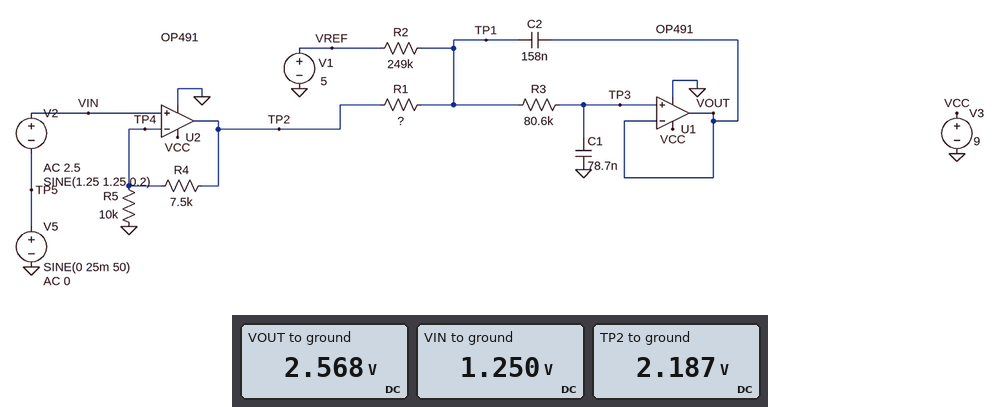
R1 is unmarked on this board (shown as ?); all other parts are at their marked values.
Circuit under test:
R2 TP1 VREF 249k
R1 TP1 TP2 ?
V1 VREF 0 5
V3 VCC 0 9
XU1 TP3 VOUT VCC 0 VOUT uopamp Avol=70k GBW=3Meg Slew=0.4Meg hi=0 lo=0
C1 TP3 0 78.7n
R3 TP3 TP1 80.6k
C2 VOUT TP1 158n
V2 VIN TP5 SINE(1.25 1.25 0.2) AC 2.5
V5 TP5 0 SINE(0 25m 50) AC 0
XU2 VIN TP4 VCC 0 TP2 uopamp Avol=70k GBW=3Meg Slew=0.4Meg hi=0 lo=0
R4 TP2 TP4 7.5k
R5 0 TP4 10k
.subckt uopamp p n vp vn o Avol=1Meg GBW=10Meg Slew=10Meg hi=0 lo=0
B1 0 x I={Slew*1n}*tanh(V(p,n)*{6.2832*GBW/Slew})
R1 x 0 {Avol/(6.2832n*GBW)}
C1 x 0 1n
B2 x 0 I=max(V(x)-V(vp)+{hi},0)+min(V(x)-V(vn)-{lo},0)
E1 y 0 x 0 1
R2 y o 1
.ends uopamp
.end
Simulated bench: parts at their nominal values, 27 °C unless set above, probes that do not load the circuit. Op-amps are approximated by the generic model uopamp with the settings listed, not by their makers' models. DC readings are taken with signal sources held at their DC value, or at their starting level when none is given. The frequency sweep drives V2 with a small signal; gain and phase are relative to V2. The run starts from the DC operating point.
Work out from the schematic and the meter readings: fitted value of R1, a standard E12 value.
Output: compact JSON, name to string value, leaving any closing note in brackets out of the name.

{"fitted value of R1, a standard E12 value": "39 kΩ"}
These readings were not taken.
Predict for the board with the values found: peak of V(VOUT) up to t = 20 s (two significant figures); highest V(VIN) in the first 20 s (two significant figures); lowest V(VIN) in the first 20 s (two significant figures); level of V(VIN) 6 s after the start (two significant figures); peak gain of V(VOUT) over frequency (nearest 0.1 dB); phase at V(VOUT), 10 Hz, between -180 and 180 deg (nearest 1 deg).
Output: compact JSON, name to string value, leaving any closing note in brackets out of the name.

{"peak of V(VOUT) up to t = 20 s": "4.5 V", "highest V(VIN) in the first 20 s": "2.5 V", "lowest V(VIN) in the first 20 s": "-25 mV", "level of V(VIN) 6 s after the start": "2.4 V", "peak gain of V(VOUT) over frequency": "3.6 dB", "phase at V(VOUT), 10 Hz, between -180 and 180 deg": "-33 deg"}
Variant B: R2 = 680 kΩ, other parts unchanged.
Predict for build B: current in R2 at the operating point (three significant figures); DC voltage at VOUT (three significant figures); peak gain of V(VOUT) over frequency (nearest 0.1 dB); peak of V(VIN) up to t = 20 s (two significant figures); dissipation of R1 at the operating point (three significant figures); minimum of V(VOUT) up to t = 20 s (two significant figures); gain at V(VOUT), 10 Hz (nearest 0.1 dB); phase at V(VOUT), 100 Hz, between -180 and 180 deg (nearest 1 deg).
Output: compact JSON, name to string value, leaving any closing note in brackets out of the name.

{"current in R2 at the operating point": "3.91 µA", "DC voltage at VOUT": "2.34 V", "peak gain of V(VOUT) over frequency": "4.4 dB", "peak of V(VIN) up to t = 20 s": "2.5 V", "dissipation of R1 at the operating point": "597 nW", "minimum of V(VOUT) up to t = 20 s": "280 mV", "gain at V(VOUT), 10 Hz": "4.1 dB", "phase at V(VOUT), 100 Hz, between -180 and 180 deg": "-157 deg"}
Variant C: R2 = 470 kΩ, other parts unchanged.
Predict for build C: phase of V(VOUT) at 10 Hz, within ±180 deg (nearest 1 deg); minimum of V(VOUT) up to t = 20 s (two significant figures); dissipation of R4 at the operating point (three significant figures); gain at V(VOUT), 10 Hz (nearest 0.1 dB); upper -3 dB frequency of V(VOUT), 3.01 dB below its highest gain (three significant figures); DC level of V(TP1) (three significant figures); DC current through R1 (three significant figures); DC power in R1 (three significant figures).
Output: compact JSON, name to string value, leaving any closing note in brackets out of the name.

{"phase of V(VOUT) at 10 Hz, within ±180 deg": "-34 deg", "minimum of V(VOUT) up to t = 20 s": "390 mV", "dissipation of R4 at the operating point": "117 µW", "gain at V(VOUT), 10 Hz": "3.9 dB", "upper -3 dB frequency of V(VOUT), 3.01 dB below its highest gain": "24.4 Hz", "DC level of V(TP1)": "2.40 V", "DC current through R1": "5.53 µA", "DC power in R1": "1.19 µW"}
